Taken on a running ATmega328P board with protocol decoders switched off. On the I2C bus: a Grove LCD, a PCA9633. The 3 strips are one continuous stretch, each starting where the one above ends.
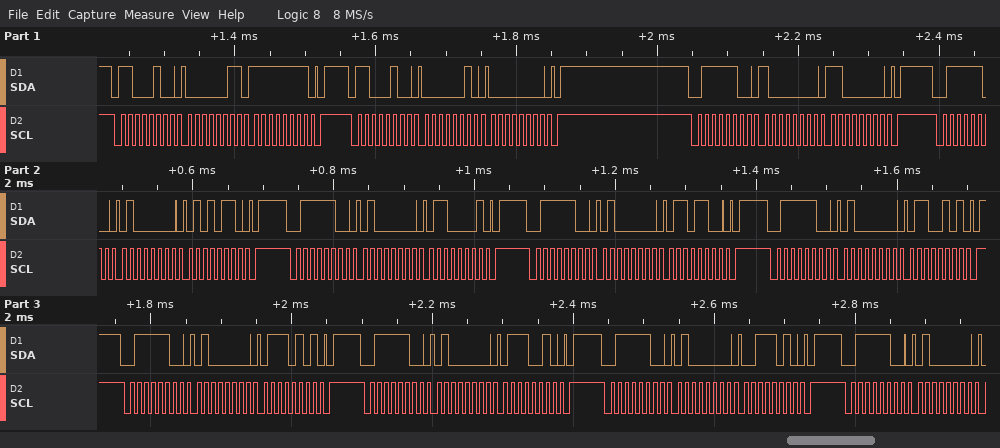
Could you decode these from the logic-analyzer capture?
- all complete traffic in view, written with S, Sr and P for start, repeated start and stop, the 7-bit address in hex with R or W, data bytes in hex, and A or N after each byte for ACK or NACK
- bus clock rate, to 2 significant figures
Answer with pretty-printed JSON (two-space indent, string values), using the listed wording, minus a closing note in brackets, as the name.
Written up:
{
  "all complete traffic in view, written with S, Sr and P for start, repeated start and stop, the 7-bit address in hex with R or W, data bytes in hex, and A or N after each byte for ACK or NACK": "S 62W A 03 A FF A P S 62W A 02 A 00 A P S 3EW A 80 A C0 A P S 3EW A 40 A 56 A P S 3EW A 40 A 61 A P S 3EW A 40 A 6C A P S 3EW A 40 A 65 A P S 3EW A 40 A 75 A P S 3EW A 40 A 72 A P S 3EW A 40 A 3A A P S 3EW A 40 A",
  "bus clock rate, to 2 significant figures": "100 kHz"
}
